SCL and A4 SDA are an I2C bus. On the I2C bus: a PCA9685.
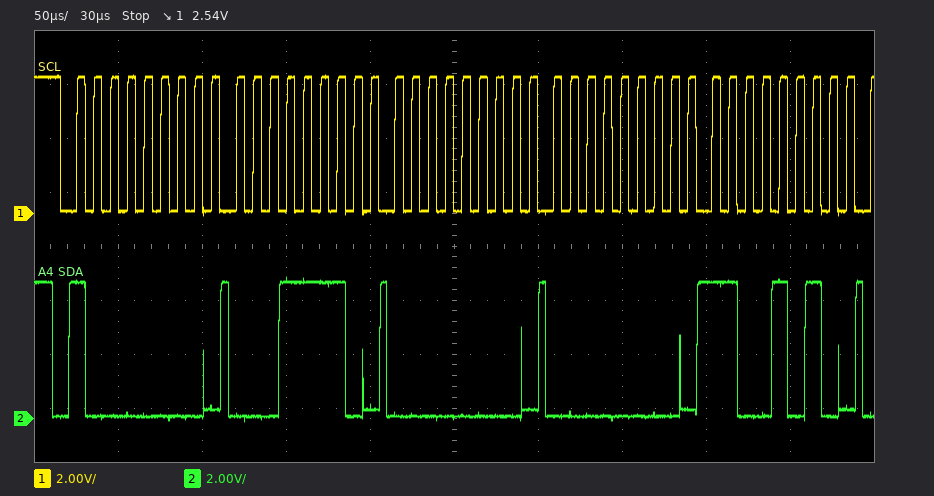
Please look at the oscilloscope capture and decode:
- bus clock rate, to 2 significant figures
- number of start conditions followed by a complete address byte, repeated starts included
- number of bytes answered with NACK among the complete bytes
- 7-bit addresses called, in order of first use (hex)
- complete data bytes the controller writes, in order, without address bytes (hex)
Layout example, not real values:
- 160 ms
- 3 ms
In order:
- 100 kHz
- 1
- 0
- 0x40
- 1E 00 00 CA
